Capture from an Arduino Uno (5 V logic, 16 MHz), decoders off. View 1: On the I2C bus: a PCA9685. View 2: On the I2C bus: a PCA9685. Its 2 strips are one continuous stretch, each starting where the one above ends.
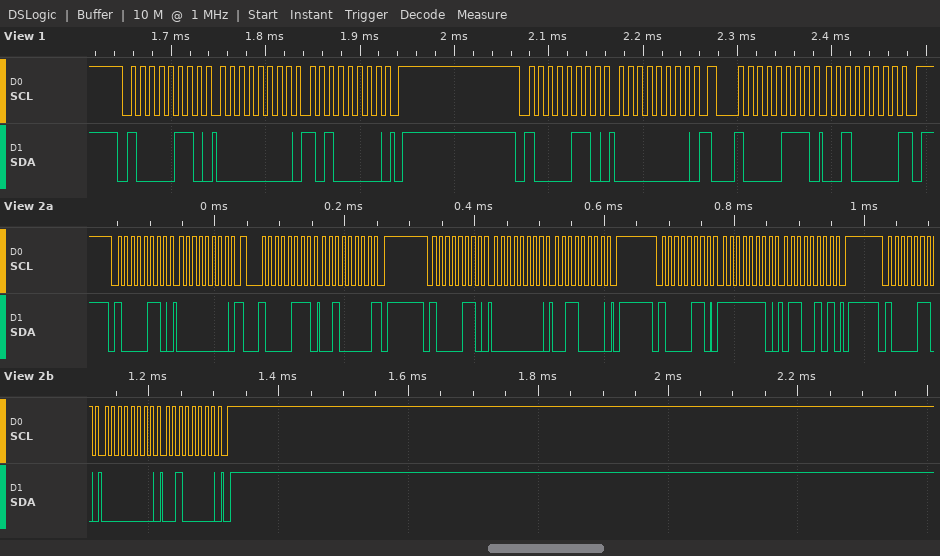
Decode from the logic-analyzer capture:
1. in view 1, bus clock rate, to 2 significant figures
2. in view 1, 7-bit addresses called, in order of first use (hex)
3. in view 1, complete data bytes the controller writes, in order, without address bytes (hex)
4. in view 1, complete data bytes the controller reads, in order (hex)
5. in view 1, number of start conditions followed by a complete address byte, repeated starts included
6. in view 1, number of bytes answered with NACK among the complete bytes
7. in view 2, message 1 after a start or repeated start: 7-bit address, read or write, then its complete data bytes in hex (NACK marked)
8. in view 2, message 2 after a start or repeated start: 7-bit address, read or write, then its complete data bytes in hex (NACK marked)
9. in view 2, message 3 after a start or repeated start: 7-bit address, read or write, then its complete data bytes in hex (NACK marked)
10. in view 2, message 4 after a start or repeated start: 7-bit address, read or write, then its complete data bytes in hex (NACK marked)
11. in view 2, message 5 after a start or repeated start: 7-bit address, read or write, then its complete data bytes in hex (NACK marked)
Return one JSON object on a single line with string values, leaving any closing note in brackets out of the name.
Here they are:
{"in view 1, bus clock rate, to 2 significant figures": "100 kHz", "in view 1, 7-bit addresses called, in order of first use": "0x43", "in view 1, complete data bytes the controller writes, in order, without address bytes": "00 A0 00", "in view 1, complete data bytes the controller reads, in order": "20", "in view 1, number of start conditions followed by a complete address byte, repeated starts included": "3", "in view 1, number of bytes answered with NACK among the complete bytes": "1", "in view 2, message 1 after a start or repeated start: 7-bit address, read or write, then its complete data bytes in hex": "0x43 write: 00", "in view 2, message 2 after a start or repeated start: 7-bit address, read or write, then its complete data bytes in hex": "0x43 read: 20 NACK", "in view 2, message 3 after a start or repeated start: 7-bit address, read or write, then its complete data bytes in hex": "0x43 write: 00 30", "in view 2, message 4 after a start or repeated start: 7-bit address, read or write, then its complete data bytes in hex": "0x43 write: FE 65", "in view 2, message 5 after a start or repeated start: 7-bit address, read or write, then its complete data bytes in hex": "0x43 write: 00 20"}
